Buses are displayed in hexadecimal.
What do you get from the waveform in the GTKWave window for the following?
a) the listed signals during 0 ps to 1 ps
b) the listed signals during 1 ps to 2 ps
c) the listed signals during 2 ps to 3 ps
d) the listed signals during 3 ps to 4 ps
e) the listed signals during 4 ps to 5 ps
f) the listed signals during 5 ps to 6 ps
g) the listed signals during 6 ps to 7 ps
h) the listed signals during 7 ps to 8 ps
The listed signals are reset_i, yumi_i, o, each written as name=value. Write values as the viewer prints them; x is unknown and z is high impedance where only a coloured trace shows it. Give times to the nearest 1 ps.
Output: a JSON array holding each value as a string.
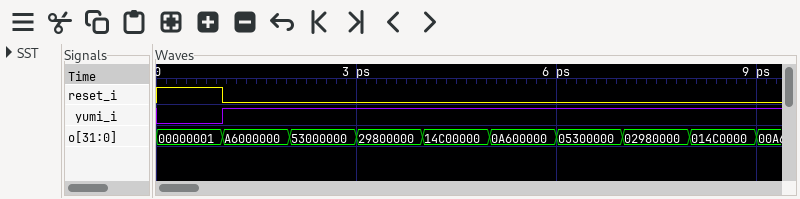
["reset_i=1, yumi_i=0, o=00000001", "reset_i=0, yumi_i=1, o=A6000000", "reset_i=0, yumi_i=1, o=53000000", "reset_i=0, yumi_i=1, o=29800000", "reset_i=0, yumi_i=1, o=14C00000", "reset_i=0, yumi_i=1, o=0A600000", "reset_i=0, yumi_i=1, o=05300000", "reset_i=0, yumi_i=1, o=02980000"]
